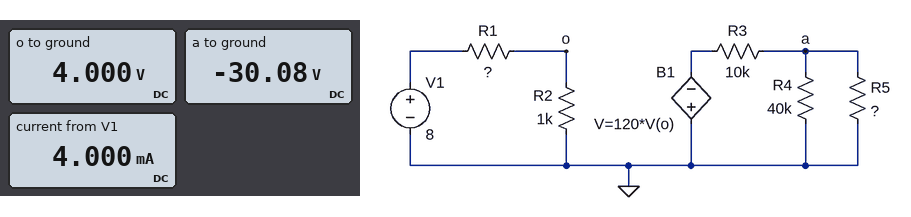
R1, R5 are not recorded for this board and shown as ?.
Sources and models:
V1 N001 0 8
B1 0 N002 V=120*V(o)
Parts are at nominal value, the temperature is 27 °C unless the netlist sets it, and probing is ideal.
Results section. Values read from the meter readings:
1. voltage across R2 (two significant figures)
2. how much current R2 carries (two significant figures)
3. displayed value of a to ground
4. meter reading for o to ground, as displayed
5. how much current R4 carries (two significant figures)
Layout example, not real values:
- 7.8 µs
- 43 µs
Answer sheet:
- 4.0 V
- 4.0 mA
- -30.08 V
- 4.000 V
- 750 µA
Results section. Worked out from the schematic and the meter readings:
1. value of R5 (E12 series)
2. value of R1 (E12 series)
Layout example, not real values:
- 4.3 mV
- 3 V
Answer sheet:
- 680 Ω
- 1 kΩ
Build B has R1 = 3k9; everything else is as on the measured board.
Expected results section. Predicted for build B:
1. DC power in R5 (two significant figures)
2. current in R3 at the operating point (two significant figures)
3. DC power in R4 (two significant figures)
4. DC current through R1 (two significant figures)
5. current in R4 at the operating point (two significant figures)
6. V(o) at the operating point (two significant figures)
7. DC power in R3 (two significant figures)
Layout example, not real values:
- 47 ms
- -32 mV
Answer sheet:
- 220 mW
- 18 mA
- 3.8 mW
- 1.6 mA
- 310 µA
- 1.6 V
- 3.4 W
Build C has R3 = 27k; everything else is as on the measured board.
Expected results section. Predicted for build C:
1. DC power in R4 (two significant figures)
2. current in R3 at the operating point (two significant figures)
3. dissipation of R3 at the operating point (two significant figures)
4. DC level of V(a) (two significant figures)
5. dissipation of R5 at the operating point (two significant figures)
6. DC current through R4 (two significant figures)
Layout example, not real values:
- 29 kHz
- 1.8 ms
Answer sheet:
- 3.4 mW
- 17 mA
- 8.1 W
- -12 V
- 200 mW
- 290 µA
